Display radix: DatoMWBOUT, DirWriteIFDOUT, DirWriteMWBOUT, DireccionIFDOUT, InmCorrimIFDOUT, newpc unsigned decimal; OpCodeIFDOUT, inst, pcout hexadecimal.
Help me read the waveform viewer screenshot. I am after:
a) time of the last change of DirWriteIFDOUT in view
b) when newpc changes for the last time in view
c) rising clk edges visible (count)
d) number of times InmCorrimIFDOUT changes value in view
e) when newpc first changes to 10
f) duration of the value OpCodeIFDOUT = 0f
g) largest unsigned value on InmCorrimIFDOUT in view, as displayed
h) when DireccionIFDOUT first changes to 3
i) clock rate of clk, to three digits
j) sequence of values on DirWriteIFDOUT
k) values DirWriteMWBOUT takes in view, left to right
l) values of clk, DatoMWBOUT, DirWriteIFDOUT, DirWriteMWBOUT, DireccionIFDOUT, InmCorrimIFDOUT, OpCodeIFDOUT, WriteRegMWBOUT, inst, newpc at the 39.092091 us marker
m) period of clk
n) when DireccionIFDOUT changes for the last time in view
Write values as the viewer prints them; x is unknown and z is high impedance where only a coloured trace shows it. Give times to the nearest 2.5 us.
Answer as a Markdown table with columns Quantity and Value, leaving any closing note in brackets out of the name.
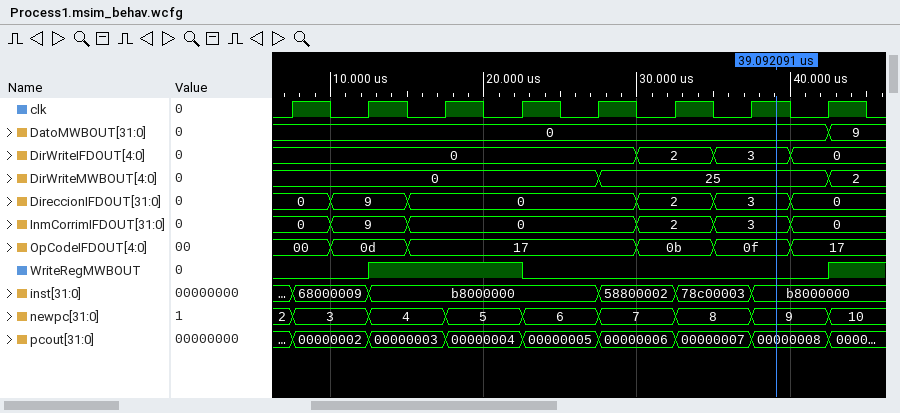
| Quantity | Value |
|---|---|
| time of the last change of DirWriteIFDOUT in view | 40 us |
| when newpc changes for the last time in view | 42.5 us |
| rising clk edges visible | 8 |
| number of times InmCorrimIFDOUT changes value in view | 5 |
| when newpc first changes to 10 | 42.5 us |
| duration of the value OpCodeIFDOUT = 0f | 5 us |
| largest unsigned value on InmCorrimIFDOUT in view, as displayed | 9 |
| when DireccionIFDOUT first changes to 3 | 35 us |
| clock rate of clk, to three digits | 200 kHz |
| sequence of values on DirWriteIFDOUT | 0, 2, 3, 0 |
| values DirWriteMWBOUT takes in view, left to right | 0, 25, 2 |
| values of clk, DatoMWBOUT, DirWriteIFDOUT, DirWriteMWBOUT, DireccionIFDOUT, InmCorrimIFDOUT, OpCodeIFDOUT, WriteRegMWBOUT, inst, newpc at the 39.092091 us marker | clk=1, DatoMWBOUT=0, DirWriteIFDOUT=3, DirWriteMWBOUT=25, DireccionIFDOUT=3, InmCorrimIFDOUT=3, OpCodeIFDOUT=0f, WriteRegMWBOUT=0, inst=b8000000, newpc=9 |
| period of clk | 5 us |
| when DireccionIFDOUT changes for the last time in view | 40 us |
